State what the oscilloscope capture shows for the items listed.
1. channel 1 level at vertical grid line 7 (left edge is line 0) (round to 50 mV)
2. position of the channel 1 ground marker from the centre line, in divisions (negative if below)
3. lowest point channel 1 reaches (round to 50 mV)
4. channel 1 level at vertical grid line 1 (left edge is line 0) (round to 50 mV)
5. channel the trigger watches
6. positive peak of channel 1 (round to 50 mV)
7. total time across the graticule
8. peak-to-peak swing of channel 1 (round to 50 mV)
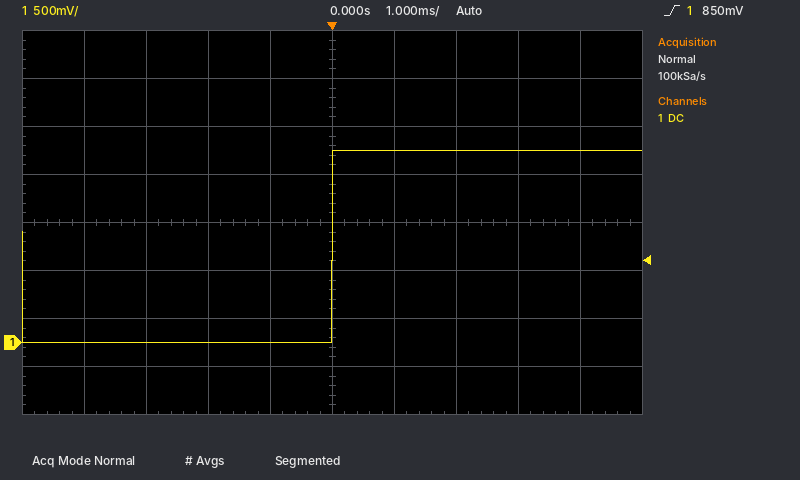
2.00 V
-2.5 div
0 mV
0 mV
channel 1
2.00 V
10 ms
2.00 V
